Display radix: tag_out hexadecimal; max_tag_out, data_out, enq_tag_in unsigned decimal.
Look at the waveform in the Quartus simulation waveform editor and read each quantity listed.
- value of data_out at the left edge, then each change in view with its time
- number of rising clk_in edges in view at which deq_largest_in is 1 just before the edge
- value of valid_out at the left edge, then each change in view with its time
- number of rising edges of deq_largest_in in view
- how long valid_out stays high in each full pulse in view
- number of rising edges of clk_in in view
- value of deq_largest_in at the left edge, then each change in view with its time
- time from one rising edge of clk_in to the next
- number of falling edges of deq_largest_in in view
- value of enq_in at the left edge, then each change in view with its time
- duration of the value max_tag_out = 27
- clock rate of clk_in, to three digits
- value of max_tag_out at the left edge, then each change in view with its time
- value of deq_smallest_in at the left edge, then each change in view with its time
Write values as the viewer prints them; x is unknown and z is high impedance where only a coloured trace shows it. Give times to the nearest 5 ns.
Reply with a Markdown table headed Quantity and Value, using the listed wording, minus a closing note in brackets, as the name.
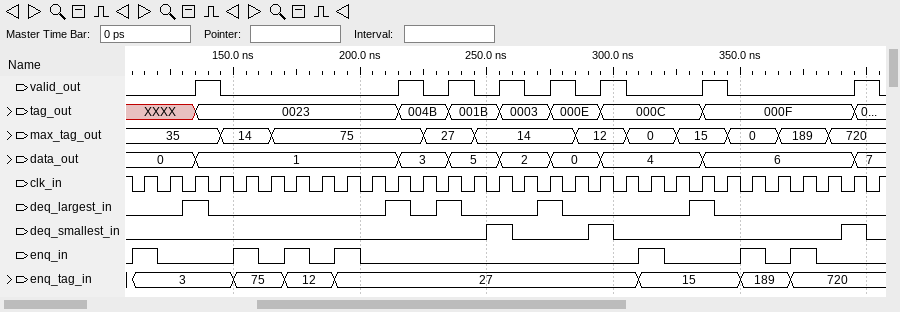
| Quantity | Value |
|---|---|
| value of data_out at the left edge, then each change in view with its time | 0, 1 at 135 ns, 3 at 215 ns, 5 at 235 ns, 2 at 255 ns, 0 at 275 ns, 4 at 295 ns, 6 at 335 ns, 7 at 395 ns |
| number of rising clk_in edges in view at which deq_largest_in is 1 just before the edge | 5 |
| value of valid_out at the left edge, then each change in view with its time | 0, 1 at 135 ns, 0 at 145 ns, 1 at 215 ns, 0 at 225 ns, 1 at 235 ns, 0 at 245 ns, 1 at 255 ns, 0 at 265 ns, 1 at 275 ns, 0 at 285 ns, 1 at 295 ns, 0 at 305 ns, 1 at 335 ns, 0 at 345 ns, 1 at 395 ns, 0 at 405 ns |
| number of rising edges of deq_largest_in in view | 5 |
| how long valid_out stays high in each full pulse in view | 10 ns, 10 ns, 10 ns, 10 ns, 10 ns, 10 ns, 10 ns, 10 ns |
| number of rising edges of clk_in in view | 30 |
| value of deq_largest_in at the left edge, then each change in view with its time | 0, 1 at 130 ns, 0 at 140 ns, 1 at 210 ns, 0 at 220 ns, 1 at 230 ns, 0 at 240 ns, 1 at 270 ns, 0 at 280 ns, 1 at 330 ns, 0 at 340 ns |
| time from one rising edge of clk_in to the next | 10 ns |
| number of falling edges of deq_largest_in in view | 5 |
| value of enq_in at the left edge, then each change in view with its time | 0, 1 at 110 ns, 0 at 120 ns, 1 at 150 ns, 0 at 160 ns, 1 at 170 ns, 0 at 180 ns, 1 at 190 ns, 0 at 200 ns, 1 at 310 ns, 0 at 320 ns, 1 at 350 ns, 0 at 360 ns, 1 at 370 ns, 0 at 380 ns |
| duration of the value max_tag_out = 27 | 20 ns |
| clock rate of clk_in, to three digits | 100 MHz |
| value of max_tag_out at the left edge, then each change in view with its time | 35, 14 at 145 ns, 75 at 165 ns, 27 at 225 ns, 14 at 245 ns, 12 at 285 ns, 0 at 305 ns, 15 at 325 ns, 0 at 345 ns, 189 at 365 ns, 720 at 385 ns |
| value of deq_smallest_in at the left edge, then each change in view with its time | 0, 1 at 250 ns, 0 at 260 ns, 1 at 290 ns, 0 at 300 ns, 1 at 390 ns, 0 at 400 ns |
